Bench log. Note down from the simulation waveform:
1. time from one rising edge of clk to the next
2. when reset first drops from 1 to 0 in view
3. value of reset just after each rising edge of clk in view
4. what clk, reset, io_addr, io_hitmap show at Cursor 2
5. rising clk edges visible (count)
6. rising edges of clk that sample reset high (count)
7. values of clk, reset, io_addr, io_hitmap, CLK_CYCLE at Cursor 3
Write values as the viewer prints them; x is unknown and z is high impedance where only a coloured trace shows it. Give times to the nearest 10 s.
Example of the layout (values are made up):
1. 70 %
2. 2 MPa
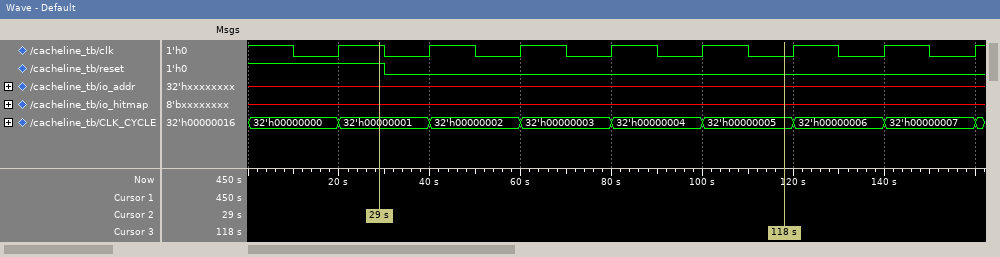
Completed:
1. 20 s
2. 30 s
3. 1 0 0 0 0 0 0 0
4. clk=1, reset=1, io_addr=x, io_hitmap=x
5. 8
6. 1
7. clk=0, reset=0, io_addr=x, io_hitmap=x, CLK_CYCLE=32'h00000005
